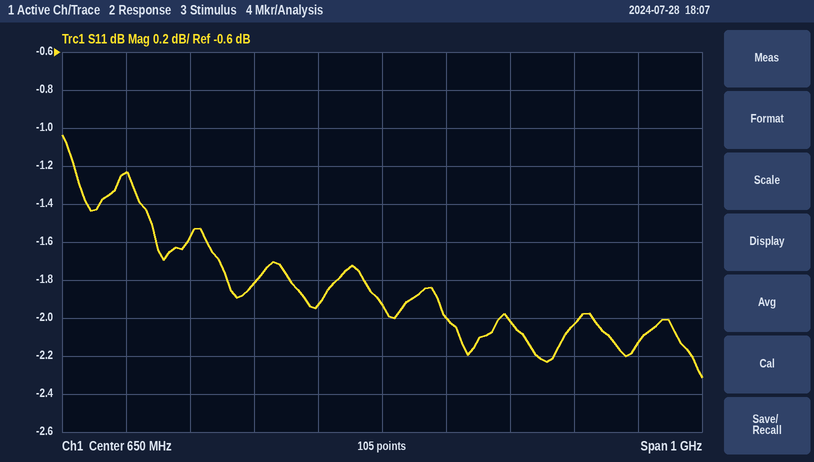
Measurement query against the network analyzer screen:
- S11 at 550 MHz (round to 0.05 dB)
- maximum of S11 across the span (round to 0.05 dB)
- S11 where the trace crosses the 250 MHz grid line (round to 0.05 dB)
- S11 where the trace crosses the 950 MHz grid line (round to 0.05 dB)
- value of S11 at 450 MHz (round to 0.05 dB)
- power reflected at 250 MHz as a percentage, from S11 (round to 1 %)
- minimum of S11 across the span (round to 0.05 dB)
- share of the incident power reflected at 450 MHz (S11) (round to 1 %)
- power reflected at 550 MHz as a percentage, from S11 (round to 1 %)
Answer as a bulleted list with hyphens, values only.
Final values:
- -1.95 dB
- -1.05 dB
- -1.25 dB
- -2.05 dB
- -1.80 dB
- 75 %
- -2.30 dB
- 66 %
- 64 %
